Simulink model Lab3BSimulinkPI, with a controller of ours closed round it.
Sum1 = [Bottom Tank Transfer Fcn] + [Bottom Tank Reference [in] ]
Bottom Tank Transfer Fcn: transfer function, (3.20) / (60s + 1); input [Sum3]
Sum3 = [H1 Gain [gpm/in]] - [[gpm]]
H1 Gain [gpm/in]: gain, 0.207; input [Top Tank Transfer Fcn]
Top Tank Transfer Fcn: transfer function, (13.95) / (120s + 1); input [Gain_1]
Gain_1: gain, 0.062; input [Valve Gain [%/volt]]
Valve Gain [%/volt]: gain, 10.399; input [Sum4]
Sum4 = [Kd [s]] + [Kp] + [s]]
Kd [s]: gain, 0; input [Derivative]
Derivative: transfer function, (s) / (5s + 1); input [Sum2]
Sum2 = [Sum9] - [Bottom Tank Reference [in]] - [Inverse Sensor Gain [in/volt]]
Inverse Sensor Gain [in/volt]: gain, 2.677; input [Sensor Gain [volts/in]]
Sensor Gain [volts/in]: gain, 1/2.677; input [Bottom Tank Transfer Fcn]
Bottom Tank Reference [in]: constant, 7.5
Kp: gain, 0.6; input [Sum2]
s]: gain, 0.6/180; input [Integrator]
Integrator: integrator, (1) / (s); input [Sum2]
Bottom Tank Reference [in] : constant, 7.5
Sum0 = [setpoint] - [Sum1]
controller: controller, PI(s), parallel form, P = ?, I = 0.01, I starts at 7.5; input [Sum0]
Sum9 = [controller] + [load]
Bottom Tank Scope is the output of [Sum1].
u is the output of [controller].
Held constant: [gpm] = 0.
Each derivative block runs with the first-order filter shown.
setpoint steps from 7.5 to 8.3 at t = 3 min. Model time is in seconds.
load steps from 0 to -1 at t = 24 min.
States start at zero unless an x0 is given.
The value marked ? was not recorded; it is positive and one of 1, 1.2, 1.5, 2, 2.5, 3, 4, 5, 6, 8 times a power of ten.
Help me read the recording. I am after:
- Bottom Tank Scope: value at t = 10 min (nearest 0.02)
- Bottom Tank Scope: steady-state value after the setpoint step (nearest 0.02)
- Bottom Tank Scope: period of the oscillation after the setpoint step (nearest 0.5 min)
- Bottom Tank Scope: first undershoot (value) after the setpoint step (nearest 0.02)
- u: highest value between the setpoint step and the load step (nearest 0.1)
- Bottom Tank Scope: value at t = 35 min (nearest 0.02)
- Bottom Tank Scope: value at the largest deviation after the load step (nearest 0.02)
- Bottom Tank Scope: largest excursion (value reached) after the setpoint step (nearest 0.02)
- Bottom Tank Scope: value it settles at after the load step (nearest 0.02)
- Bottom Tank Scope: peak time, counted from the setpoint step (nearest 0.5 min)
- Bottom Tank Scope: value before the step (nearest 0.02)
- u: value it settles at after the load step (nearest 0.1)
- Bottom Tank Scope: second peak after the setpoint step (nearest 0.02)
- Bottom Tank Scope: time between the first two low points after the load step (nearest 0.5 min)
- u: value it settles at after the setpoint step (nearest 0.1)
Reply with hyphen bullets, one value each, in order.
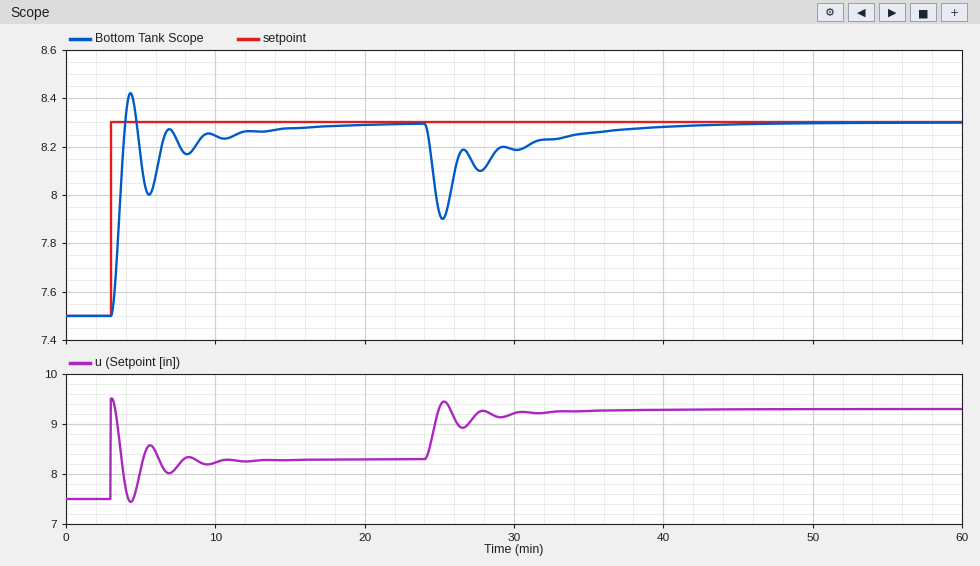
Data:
- 8.24
- 8.30
- 2.5 min
- 8.00
- 9.5
- 8.26
- 7.90
- 8.42
- 8.30
- 1.5 min
- 7.50
- 9.3
- 8.28
- 2.5 min
- 8.3
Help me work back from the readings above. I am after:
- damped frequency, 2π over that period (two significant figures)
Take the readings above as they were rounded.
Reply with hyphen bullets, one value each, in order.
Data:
- 2.5 rad/min
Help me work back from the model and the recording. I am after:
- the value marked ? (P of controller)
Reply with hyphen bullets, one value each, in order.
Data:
- 2.5
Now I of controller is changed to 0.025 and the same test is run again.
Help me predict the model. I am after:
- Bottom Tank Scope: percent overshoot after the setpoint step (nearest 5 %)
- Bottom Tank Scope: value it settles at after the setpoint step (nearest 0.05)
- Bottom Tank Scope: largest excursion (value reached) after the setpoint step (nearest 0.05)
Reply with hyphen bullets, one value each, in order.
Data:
- 30 %
- 8.30
- 8.55
